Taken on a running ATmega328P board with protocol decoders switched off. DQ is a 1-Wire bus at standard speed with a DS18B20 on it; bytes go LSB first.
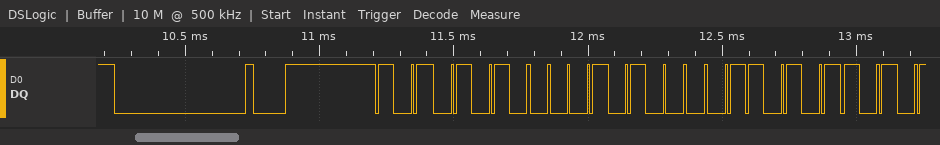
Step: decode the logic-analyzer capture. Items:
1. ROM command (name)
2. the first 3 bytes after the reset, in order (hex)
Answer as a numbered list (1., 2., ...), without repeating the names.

1. Match ROM
2. 55 28 AC
